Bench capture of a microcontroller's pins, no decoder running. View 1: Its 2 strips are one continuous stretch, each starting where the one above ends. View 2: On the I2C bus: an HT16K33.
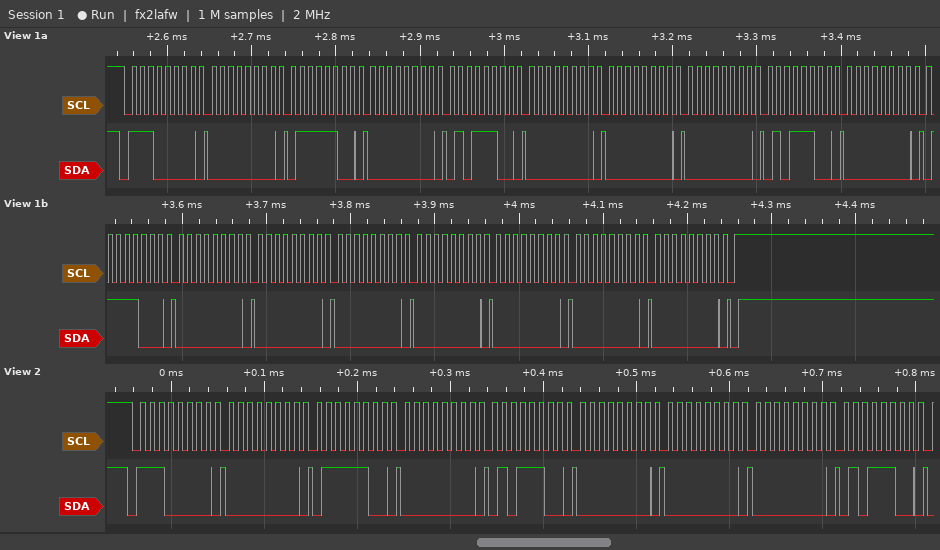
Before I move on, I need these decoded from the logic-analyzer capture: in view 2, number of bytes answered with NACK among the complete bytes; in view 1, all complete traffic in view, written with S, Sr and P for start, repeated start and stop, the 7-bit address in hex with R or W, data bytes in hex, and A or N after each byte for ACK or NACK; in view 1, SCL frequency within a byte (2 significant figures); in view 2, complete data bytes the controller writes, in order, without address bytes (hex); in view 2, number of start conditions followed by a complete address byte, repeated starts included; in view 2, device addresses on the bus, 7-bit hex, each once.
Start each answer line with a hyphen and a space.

- 0
- S 70W A 00 A 7C A 00 A 5C A 00 A 00 A 00 A 5C A 00 A 78 A 00 A 00 A 00 A 00 A 00 A 00 A 00 A P
- 100 kHz
- 00 7C 00 5C 00 00 00 5C
- 1
- 0x70
